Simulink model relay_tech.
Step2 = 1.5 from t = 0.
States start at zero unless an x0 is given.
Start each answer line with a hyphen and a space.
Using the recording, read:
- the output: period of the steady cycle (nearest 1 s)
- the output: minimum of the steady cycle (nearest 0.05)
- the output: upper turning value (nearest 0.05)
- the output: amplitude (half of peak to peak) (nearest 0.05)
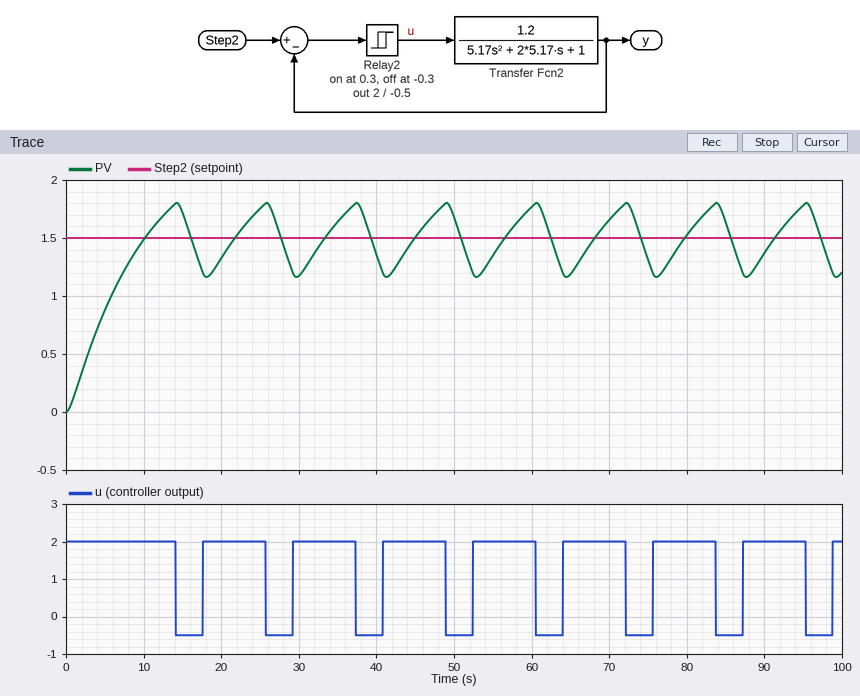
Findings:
- 12 s
- 1.15
- 1.80
- 0.30
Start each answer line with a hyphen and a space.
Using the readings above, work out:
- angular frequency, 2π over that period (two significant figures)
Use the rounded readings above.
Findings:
- 0.52 rad/s
